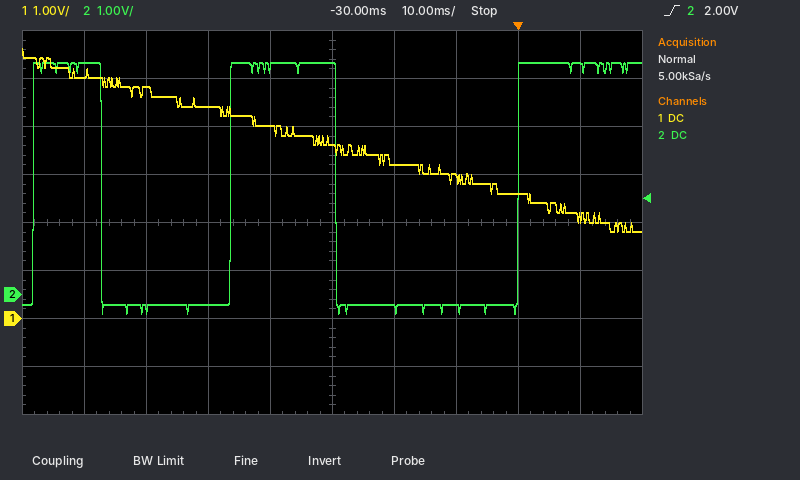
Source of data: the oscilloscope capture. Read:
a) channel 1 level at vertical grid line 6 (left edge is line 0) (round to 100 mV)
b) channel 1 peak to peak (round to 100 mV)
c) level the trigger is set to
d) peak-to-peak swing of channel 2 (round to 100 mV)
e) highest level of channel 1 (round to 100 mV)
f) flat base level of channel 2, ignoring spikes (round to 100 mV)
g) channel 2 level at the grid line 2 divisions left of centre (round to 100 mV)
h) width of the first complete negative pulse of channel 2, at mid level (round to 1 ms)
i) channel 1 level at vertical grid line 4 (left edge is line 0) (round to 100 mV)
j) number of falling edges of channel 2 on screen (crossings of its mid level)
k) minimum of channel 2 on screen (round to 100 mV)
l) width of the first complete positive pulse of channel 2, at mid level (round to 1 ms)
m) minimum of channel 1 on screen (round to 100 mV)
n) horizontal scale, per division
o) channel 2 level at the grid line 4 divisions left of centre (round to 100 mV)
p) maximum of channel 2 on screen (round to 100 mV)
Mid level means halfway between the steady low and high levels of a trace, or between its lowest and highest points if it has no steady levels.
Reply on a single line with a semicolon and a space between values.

3.2 V; 3.8 V; 2.00 V; 5.2 V; 5.6 V; -200 mV; -200 mV; 21 ms; 4.0 V; 2; -400 mV; 11 ms; 1.8 V; 10 ms; 4.8 V; 4.8 V
